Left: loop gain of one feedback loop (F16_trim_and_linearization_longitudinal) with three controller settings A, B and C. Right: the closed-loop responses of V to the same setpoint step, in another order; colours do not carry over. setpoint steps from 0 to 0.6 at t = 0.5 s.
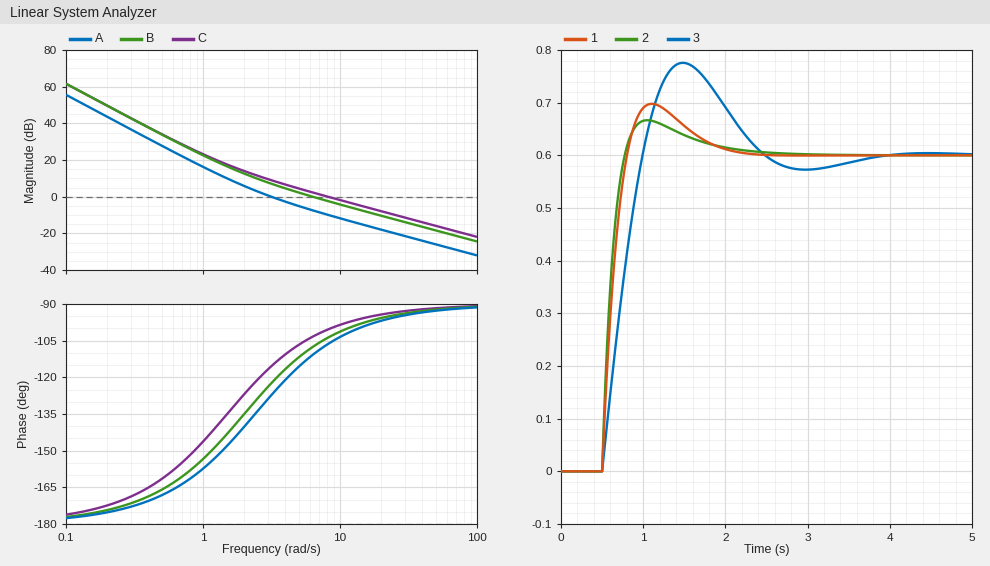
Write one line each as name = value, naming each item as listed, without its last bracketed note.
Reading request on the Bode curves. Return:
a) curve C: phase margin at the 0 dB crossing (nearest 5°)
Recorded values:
curve C: phase margin at the 0 dB crossing = 80°
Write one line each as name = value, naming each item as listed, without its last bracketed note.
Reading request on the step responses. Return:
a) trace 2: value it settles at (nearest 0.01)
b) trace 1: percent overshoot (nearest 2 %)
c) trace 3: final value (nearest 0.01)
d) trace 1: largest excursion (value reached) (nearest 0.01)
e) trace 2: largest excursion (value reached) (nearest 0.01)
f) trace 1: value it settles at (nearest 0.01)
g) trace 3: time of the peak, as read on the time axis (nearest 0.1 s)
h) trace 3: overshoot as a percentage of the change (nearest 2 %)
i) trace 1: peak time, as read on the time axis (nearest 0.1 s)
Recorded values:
trace 2: value it settles at = 0.60
trace 1: percent overshoot = 16 %
trace 3: final value = 0.60
trace 1: largest excursion (value reached) = 0.70
trace 2: largest excursion (value reached) = 0.67
trace 1: value it settles at = 0.60
trace 3: time of the peak, as read on the time axis = 1.5 s
trace 3: overshoot as a percentage of the change = 30 %
trace 1: peak time, as read on the time axis = 1.1 s
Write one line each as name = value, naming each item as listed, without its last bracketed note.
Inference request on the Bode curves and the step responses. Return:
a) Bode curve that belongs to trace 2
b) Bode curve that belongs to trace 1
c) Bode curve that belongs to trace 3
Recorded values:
Bode curve that belongs to trace 2 = C
Bode curve that belongs to trace 1 = B
Bode curve that belongs to trace 3 = A
